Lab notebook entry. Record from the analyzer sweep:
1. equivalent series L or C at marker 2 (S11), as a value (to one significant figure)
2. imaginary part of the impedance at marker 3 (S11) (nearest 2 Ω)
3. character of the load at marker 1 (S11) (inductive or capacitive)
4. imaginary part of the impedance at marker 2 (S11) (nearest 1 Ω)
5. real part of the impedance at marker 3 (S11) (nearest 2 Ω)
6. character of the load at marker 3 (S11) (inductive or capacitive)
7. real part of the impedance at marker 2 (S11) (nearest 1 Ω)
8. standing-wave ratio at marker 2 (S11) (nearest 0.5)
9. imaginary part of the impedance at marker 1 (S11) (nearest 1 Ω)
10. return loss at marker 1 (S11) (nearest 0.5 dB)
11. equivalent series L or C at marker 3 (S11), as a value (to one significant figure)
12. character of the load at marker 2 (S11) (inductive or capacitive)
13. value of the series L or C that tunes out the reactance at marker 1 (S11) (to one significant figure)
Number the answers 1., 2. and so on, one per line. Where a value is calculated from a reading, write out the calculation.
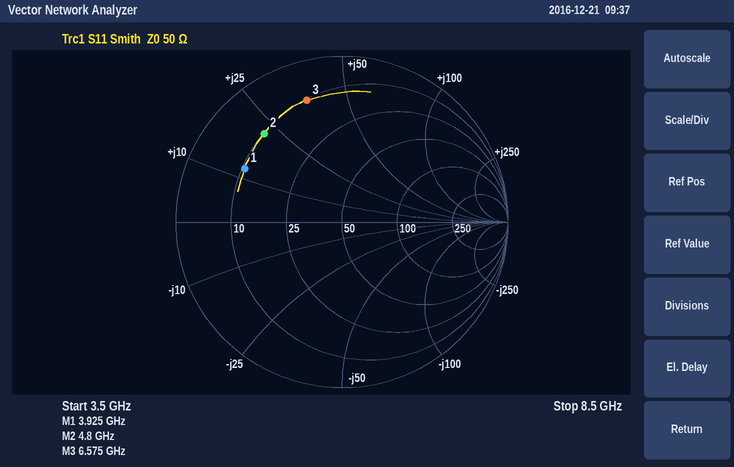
1. L = 22 Ω/(2π × 4.8 GHz) ≈ 729 pH, so 700 pH to one significant figure
2. +36 Ω
3. inductive
4. +22 Ω
5. 10 Ω
6. inductive
7. 10 Ω
8. 6.0
9. +12 Ω
10. 3.5 dB
11. L = 36 Ω/(2π × 6.575 GHz) ≈ 871 pH, so 900 pH to one significant figure
12. inductive
13. C = 1/(2π × 3.925 GHz × 12 Ω) ≈ 3 pF
